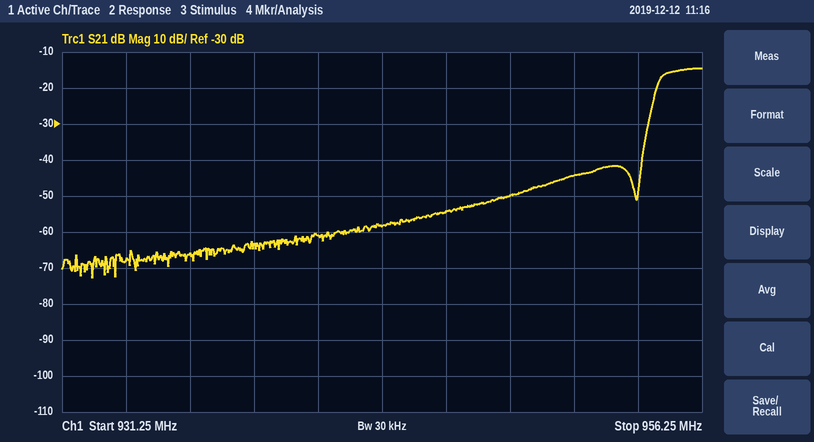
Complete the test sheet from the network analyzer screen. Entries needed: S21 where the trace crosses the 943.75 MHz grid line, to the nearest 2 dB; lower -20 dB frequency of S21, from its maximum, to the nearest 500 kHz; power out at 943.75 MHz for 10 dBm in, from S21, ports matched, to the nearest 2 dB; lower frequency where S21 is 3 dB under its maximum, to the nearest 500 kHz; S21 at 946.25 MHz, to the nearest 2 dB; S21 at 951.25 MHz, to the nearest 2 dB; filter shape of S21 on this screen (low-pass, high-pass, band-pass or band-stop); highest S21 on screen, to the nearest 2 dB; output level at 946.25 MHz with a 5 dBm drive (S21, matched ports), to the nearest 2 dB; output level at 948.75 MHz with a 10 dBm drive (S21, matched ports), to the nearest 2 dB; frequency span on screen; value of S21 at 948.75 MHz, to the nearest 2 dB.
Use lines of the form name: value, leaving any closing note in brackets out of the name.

S21 where the trace crosses the 943.75 MHz grid line, to the nearest 2 dB: -58 dB
lower -20 dB frequency of S21, from its maximum, to the nearest 500 kHz: 954.0 MHz
power out at 943.75 MHz for 10 dBm in, from S21, ports matched, to the nearest 2 dB: -48 dBm
lower frequency where S21 is 3 dB under its maximum, to the nearest 500 kHz: 954.5 MHz
S21 at 946.25 MHz, to the nearest 2 dB: -54 dB
S21 at 951.25 MHz, to the nearest 2 dB: -44 dB
filter shape of S21 on this screen: high-pass
highest S21 on screen, to the nearest 2 dB: -14 dB
output level at 946.25 MHz with a 5 dBm drive (S21, matched ports), to the nearest 2 dB: -50 dBm
output level at 948.75 MHz with a 10 dBm drive (S21, matched ports), to the nearest 2 dB: -40 dBm
frequency span on screen: 25 MHz
value of S21 at 948.75 MHz, to the nearest 2 dB: -50 dB
